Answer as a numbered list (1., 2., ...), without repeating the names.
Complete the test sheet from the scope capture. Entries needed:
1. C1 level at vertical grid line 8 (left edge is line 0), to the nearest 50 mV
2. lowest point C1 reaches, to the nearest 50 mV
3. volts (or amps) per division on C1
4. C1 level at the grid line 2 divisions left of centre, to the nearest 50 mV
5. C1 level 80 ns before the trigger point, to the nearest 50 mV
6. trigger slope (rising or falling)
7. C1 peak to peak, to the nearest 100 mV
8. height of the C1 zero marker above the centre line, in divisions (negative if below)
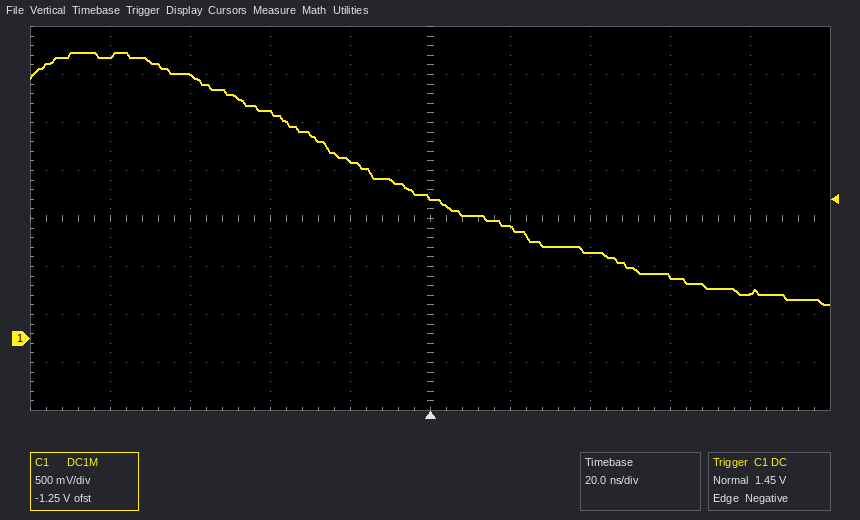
1. 650 mV
2. 350 mV
3. 500 mV
4. 2.35 V
5. 2.95 V
6. falling
7. 2.60 V
8. -2.5 div
